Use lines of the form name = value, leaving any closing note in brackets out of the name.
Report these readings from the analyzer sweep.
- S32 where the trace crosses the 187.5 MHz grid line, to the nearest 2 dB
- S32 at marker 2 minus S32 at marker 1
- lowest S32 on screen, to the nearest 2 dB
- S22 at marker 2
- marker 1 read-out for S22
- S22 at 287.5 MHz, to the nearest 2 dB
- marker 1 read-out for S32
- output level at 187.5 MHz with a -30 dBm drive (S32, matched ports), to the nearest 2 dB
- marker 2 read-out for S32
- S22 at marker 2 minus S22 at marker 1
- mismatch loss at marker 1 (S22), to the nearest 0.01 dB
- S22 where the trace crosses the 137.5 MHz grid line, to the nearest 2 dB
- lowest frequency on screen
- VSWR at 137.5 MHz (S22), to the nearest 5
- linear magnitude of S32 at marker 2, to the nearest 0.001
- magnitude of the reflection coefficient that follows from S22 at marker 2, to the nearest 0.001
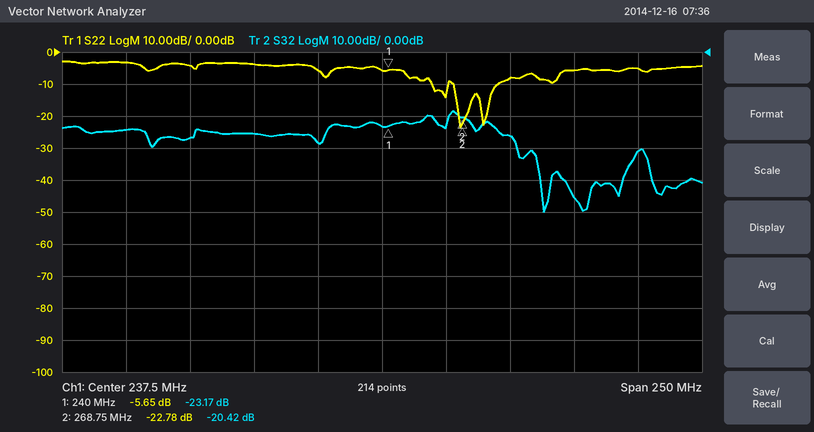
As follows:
S32 where the trace crosses the 187.5 MHz grid line, to the nearest 2 dB = -26 dB
S32 at marker 2 minus S32 at marker 1 = 2.75 dB
lowest S32 on screen, to the nearest 2 dB = -50 dB
S22 at marker 2 = -22.78 dB
marker 1 read-out for S22 = -5.65 dB
S22 at 287.5 MHz, to the nearest 2 dB = -8 dB
marker 1 read-out for S32 = -23.17 dB
output level at 187.5 MHz with a -30 dBm drive (S32, matched ports), to the nearest 2 dB = -56 dBm
marker 2 read-out for S32 = -20.42 dB
S22 at marker 2 minus S22 at marker 1 = -17.13 dB
mismatch loss at marker 1 (S22), to the nearest 0.01 dB = 1.38 dB
S22 where the trace crosses the 137.5 MHz grid line, to the nearest 2 dB = -4 dB
lowest frequency on screen = 112.5 MHz
VSWR at 137.5 MHz (S22), to the nearest 5 = 5
linear magnitude of S32 at marker 2, to the nearest 0.001 = 0.095
magnitude of the reflection coefficient that follows from S22 at marker 2, to the nearest 0.001 = 0.073
